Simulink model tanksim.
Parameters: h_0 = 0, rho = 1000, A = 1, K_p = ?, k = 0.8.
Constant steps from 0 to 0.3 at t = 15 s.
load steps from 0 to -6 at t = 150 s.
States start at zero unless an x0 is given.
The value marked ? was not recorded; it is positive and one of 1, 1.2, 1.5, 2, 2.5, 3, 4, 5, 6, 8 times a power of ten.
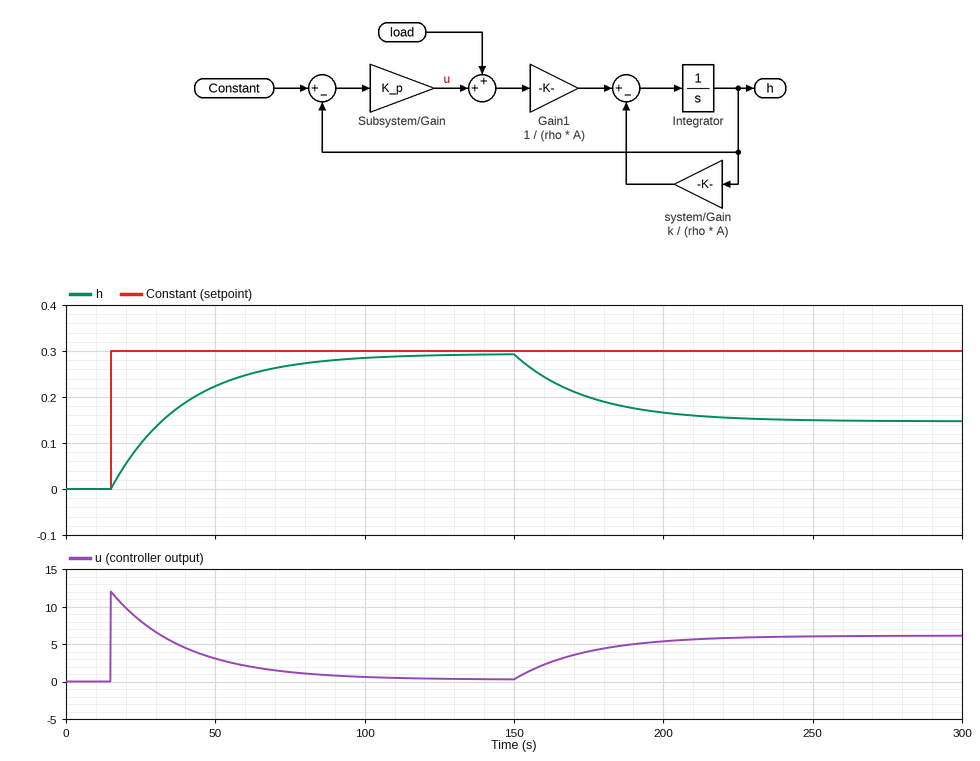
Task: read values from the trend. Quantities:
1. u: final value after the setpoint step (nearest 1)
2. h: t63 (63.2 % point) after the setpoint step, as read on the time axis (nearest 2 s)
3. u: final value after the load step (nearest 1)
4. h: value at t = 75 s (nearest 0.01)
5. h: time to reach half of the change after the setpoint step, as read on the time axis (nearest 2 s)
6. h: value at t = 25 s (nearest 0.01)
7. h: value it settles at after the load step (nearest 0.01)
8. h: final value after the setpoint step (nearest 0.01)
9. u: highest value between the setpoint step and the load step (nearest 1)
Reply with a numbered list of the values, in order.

1. 0
2. 40 s
3. 6
4. 0.27
5. 32 s
6. 0.10
7. 0.15
8. 0.29
9. 12
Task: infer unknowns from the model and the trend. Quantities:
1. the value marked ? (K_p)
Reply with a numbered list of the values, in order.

1. 40
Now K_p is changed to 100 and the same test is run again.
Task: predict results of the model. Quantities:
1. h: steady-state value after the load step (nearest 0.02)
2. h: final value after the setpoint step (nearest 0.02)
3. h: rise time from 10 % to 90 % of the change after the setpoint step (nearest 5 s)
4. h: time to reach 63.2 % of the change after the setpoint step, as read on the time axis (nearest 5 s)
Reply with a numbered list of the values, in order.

1. 0.24
2. 0.30
3. 20 s
4. 25 s
